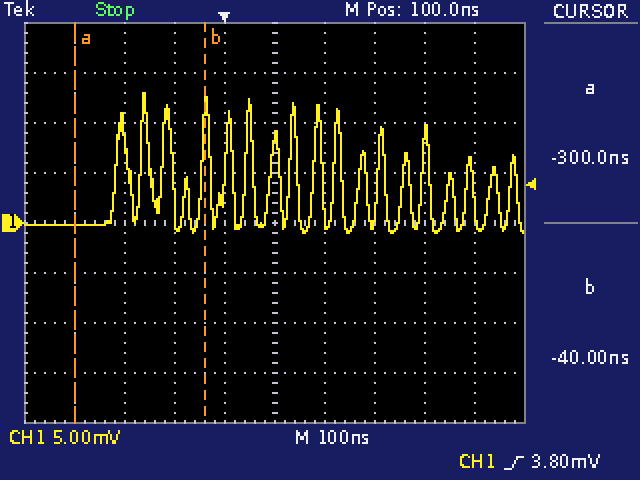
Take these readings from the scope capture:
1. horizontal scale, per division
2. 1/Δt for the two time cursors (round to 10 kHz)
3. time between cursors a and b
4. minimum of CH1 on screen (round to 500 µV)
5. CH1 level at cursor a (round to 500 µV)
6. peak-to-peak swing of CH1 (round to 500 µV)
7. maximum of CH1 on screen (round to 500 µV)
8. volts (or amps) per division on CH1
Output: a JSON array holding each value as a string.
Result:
["100 ns", "3.85 MHz", "260 ns", "-1.0 mV", "0.0 mV", "14.0 mV", "13.0 mV", "5 mV"]
